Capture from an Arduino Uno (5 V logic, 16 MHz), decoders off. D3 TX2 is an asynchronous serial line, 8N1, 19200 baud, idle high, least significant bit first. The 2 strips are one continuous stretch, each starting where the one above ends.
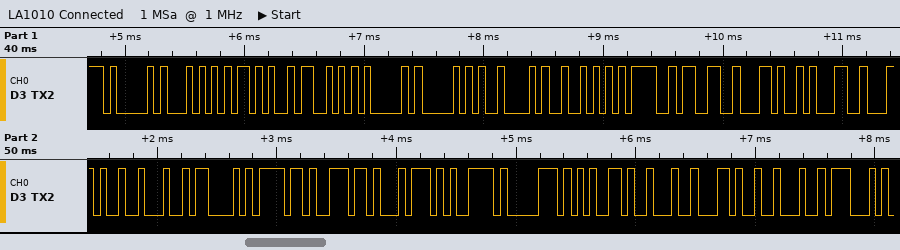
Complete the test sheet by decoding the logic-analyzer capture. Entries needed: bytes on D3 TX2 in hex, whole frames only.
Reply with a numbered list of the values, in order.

1. 41 54 2B 53 41 50 42 52 3D 33 2C 31 2C 22 43 6F 6E 74 79 70 65 22 2C 22 47
